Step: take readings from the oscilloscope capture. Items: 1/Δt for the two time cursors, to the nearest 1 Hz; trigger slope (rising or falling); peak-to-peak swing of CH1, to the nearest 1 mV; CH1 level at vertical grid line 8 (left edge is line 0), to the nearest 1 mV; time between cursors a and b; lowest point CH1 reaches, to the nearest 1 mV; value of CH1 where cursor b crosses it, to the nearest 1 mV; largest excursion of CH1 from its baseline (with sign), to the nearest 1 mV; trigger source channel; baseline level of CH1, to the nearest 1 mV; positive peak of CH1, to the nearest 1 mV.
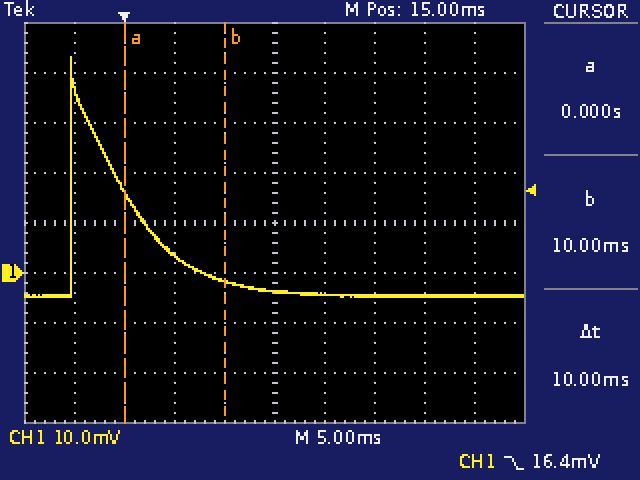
100 Hz
falling
48 mV
-5 mV
10 ms
-5 mV
-2 mV
+48 mV
CH1
-5 mV
43 mV
